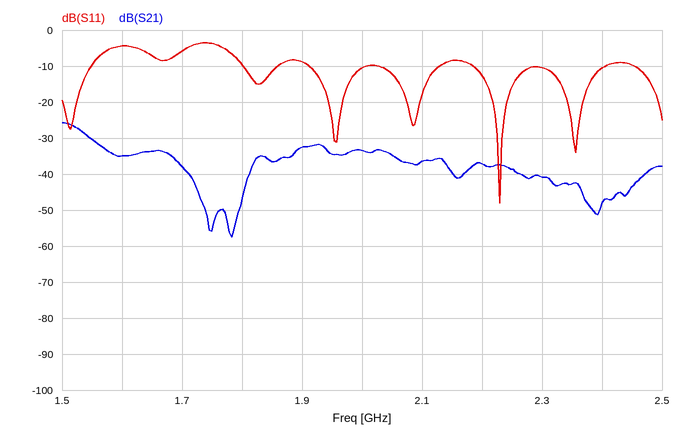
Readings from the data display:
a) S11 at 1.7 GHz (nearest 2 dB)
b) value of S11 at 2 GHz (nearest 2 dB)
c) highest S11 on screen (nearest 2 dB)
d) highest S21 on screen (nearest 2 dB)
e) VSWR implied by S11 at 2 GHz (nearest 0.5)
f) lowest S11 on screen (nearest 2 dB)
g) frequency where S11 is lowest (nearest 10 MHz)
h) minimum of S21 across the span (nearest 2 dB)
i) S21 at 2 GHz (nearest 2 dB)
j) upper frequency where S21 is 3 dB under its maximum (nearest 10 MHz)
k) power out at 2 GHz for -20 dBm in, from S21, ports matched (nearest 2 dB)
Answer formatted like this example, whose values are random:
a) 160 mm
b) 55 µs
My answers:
a) -6 dB
b) -10 dB
c) -4 dB
d) -26 dB
e) 2.0
f) -48 dB
g) 2.23 GHz
h) -58 dB
i) -34 dB
j) 1.54 GHz
k) -54 dBm
